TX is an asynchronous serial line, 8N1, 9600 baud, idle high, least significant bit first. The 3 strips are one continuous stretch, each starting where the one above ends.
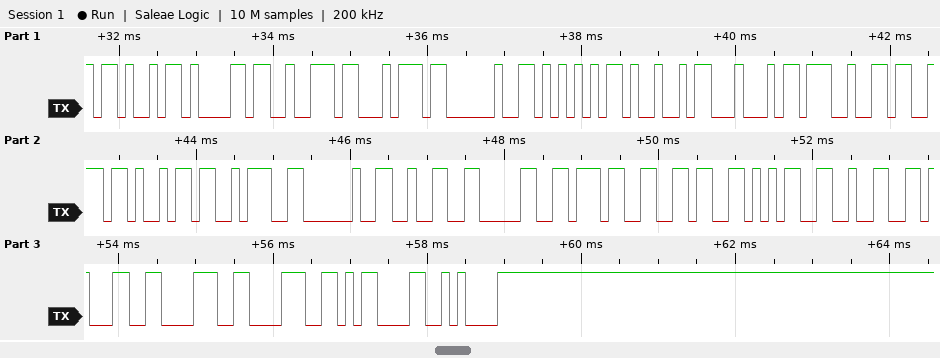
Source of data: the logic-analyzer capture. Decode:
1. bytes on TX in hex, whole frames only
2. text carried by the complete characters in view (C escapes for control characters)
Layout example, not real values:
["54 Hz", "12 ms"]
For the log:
["0x4B 0x61 0x72 0x74 0x20 0x55 0x49 0x44 0x27 0x73 0x69 0x3A 0x20 0x32 0x30 0x37 0x36 0x35 0x32 0x31 0x38 0x38 0x0D 0x0A", "\"Kart UID'si: 207652188\\r\\n\""]
